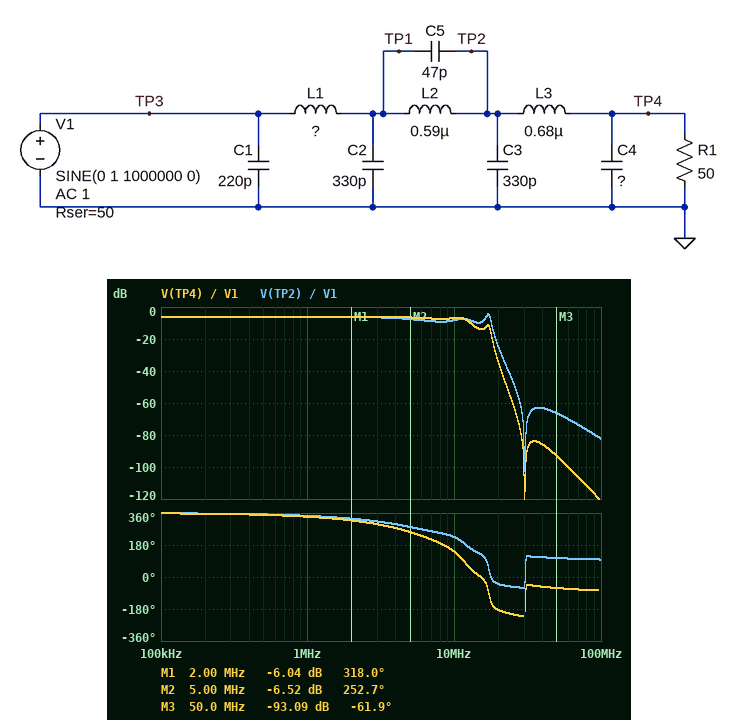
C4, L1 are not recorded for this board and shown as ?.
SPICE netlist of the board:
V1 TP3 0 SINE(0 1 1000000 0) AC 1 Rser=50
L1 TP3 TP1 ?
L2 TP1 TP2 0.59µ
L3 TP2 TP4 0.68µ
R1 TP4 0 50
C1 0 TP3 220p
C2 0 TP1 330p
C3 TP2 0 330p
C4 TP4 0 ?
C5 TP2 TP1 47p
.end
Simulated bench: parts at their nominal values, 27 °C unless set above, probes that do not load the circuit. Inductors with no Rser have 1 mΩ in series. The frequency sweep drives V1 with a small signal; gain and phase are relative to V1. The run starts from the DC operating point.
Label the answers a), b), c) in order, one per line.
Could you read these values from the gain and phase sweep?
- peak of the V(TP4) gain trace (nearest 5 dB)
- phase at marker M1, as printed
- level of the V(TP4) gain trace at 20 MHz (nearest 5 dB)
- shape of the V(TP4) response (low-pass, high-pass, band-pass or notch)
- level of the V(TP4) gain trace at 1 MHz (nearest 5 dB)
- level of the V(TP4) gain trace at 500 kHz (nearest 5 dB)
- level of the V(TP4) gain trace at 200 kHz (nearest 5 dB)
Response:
a) -5 dB
b) 318.0 deg
c) -35 dB
d) low-pass
e) -5 dB
f) -5 dB
g) -5 dB
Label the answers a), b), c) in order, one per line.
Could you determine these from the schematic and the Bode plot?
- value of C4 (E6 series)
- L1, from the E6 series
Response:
a) 330 pF
b) 1.5 µH
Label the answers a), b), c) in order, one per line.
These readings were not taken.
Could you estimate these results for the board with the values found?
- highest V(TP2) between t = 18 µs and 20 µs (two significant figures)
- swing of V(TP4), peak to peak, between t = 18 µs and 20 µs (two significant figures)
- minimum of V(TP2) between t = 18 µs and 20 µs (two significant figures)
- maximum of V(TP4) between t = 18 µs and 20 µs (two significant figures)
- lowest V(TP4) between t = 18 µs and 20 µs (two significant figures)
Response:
a) 500 mV
b) 1.0 V
c) -500 mV
d) 500 mV
e) -500 mV
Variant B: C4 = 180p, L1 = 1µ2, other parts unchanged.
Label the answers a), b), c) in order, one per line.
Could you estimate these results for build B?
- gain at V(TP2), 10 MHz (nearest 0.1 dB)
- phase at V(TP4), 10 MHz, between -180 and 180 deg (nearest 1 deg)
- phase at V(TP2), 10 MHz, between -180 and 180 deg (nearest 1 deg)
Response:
a) -6.7 dB
b) 162 deg
c) -139 deg
